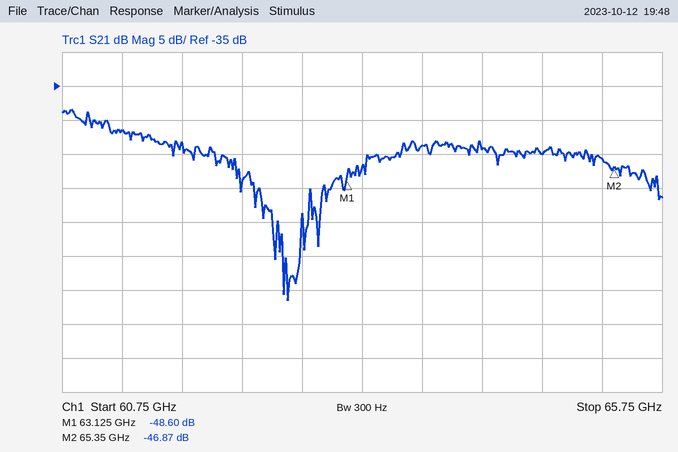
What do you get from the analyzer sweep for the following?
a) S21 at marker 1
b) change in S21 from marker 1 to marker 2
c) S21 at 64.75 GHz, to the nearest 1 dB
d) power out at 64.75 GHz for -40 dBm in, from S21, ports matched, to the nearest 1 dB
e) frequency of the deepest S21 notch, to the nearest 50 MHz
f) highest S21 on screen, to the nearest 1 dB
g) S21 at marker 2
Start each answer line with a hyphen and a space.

- -48.60 dB
- 1.73 dB
- -45 dB
- -85 dBm
- 62.65 GHz
- -38 dB
- -46.87 dB
